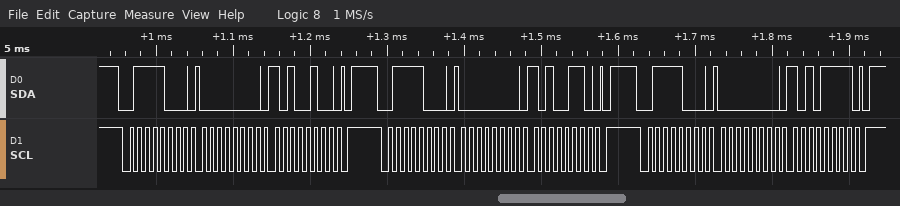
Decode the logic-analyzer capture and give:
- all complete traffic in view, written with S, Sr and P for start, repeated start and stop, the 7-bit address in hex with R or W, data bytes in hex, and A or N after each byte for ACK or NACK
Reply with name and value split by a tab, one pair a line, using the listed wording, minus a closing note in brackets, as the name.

all complete traffic in view, written with S, Sr and P for start, repeated start and stop, the 7-bit address in hex with R or W, data bytes in hex, and A or N after each byte for ACK or NACK	S 3CW A 00 A A4 A P S 3CW A 00 A A6 A P S 3CW A 00 A AF A P
